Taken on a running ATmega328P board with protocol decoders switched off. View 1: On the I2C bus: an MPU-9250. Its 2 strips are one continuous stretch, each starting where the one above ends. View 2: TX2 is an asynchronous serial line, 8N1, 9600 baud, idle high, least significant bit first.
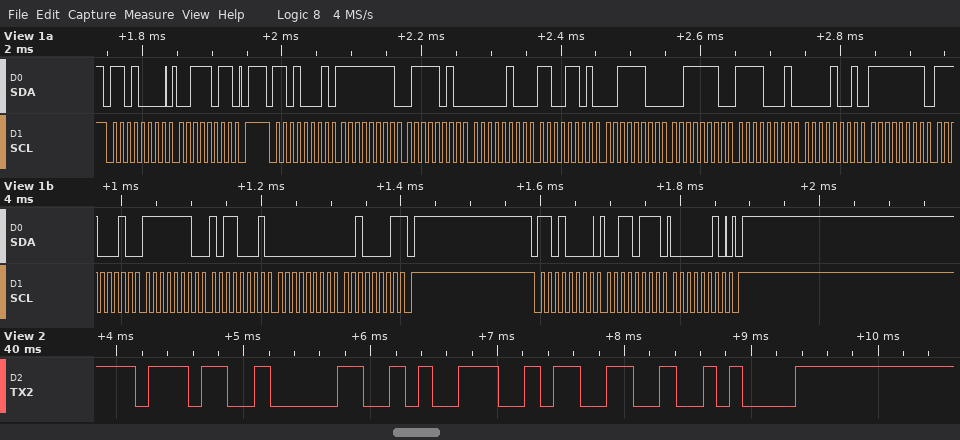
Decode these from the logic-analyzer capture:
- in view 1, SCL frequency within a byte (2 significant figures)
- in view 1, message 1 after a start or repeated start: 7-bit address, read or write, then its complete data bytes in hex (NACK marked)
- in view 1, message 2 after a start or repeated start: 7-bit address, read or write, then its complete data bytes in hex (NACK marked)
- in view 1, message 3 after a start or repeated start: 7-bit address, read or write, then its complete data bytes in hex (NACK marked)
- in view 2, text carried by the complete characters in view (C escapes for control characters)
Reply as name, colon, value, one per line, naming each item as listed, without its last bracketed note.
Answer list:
in view 1, SCL frequency within a byte: 100 kHz
in view 1, message 1 after a start or repeated start: 7-bit address, read or write, then its complete data bytes in hex: 0x68 write: 3B
in view 1, message 2 after a start or repeated start: 7-bit address, read or write, then its complete data bytes in hex: 0x68 read: FF 7A 04 CD 3C 3E F1 09 FF E2 FE B1 00 21 NACK
in view 1, message 3 after a start or repeated start: 7-bit address, read or write, then its complete data bytes in hex: 0x68 write: 37 02
in view 2, text carried by the complete characters in view: "7093\n"
